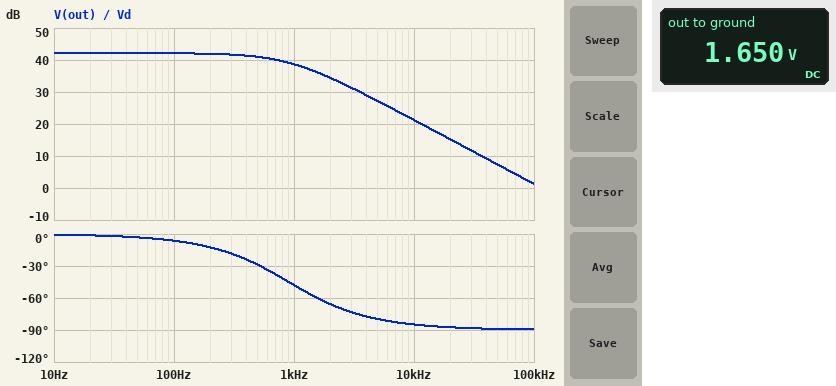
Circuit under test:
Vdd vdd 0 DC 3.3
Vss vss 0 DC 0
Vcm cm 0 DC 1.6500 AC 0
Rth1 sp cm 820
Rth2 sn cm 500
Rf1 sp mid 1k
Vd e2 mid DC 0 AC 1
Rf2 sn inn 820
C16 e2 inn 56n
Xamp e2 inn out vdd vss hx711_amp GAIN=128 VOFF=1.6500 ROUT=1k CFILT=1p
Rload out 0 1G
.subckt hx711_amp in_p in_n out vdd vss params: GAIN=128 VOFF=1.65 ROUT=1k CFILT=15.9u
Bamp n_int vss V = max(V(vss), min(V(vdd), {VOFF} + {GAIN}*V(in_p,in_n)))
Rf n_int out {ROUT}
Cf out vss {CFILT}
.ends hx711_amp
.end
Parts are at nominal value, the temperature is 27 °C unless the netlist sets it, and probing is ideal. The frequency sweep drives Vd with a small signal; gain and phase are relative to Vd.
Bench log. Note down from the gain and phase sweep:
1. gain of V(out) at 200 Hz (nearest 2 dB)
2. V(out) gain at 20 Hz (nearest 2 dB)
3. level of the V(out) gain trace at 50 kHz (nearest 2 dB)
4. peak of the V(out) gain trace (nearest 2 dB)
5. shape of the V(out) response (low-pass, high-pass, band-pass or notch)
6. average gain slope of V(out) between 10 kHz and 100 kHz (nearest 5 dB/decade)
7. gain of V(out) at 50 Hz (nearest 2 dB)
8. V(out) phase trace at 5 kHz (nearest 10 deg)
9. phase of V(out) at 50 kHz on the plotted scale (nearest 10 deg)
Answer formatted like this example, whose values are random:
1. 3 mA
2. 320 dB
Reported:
1. 42 dB
2. 42 dB
3. 8 dB
4. 42 dB
5. low-pass
6. -20 dB/decade
7. 42 dB
8. -80 deg
9. -90 deg
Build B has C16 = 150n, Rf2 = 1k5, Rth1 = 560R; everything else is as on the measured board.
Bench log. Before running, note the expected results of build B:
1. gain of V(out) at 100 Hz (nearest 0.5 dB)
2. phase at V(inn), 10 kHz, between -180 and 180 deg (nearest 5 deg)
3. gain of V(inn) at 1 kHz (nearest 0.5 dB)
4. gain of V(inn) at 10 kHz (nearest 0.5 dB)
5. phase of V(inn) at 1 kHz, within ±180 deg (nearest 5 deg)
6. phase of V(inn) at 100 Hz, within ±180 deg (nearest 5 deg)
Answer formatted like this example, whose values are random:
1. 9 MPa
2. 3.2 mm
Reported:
1. 41.5 dB
2. 0 deg
3. -5.5 dB
4. -5.0 dB
5. 15 deg
6. 70 deg
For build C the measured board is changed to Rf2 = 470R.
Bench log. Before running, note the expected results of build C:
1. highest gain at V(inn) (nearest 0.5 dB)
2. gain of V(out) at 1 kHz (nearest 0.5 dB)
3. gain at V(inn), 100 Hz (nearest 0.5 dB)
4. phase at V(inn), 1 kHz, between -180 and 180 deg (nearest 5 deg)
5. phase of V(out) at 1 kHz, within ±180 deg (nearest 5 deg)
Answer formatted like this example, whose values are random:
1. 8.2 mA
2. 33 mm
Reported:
1. -9.0 dB
2. 39.0 dB
3. -29.5 dB
4. 45 deg
5. -45 deg
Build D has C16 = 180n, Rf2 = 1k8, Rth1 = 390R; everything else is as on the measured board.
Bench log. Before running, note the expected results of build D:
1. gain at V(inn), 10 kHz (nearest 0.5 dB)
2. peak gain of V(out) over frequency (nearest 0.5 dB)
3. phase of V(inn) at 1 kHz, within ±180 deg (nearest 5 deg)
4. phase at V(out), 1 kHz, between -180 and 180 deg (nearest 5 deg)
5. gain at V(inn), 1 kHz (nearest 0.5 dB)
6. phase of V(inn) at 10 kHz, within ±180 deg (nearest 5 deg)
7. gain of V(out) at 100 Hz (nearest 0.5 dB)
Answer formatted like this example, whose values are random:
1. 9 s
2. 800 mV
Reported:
1. -4.0 dB
2. 42.0 dB
3. 15 deg
4. -75 deg
5. -4.5 dB
6. 0 deg
7. 41.5 dB
